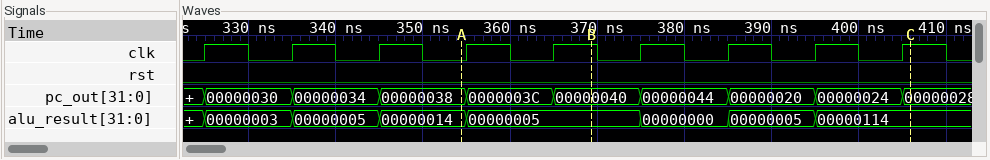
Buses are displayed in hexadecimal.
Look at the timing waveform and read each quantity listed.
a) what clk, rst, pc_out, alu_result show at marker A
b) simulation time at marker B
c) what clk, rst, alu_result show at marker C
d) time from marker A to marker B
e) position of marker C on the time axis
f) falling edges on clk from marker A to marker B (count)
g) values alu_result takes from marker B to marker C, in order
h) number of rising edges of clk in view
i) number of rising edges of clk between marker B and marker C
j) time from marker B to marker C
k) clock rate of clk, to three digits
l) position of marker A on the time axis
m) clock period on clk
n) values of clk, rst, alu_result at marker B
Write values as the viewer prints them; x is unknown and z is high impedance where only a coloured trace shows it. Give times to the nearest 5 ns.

clk=0, rst=0, pc_out=00000038, alu_result=00000014
370 ns
clk=1, rst=0, alu_result=00000114
15 ns
405 ns
1
00000005, 00000000, 00000005, 00000114
9
4
35 ns
100 MHz
355 ns
10 ns
clk=1, rst=0, alu_result=00000005
